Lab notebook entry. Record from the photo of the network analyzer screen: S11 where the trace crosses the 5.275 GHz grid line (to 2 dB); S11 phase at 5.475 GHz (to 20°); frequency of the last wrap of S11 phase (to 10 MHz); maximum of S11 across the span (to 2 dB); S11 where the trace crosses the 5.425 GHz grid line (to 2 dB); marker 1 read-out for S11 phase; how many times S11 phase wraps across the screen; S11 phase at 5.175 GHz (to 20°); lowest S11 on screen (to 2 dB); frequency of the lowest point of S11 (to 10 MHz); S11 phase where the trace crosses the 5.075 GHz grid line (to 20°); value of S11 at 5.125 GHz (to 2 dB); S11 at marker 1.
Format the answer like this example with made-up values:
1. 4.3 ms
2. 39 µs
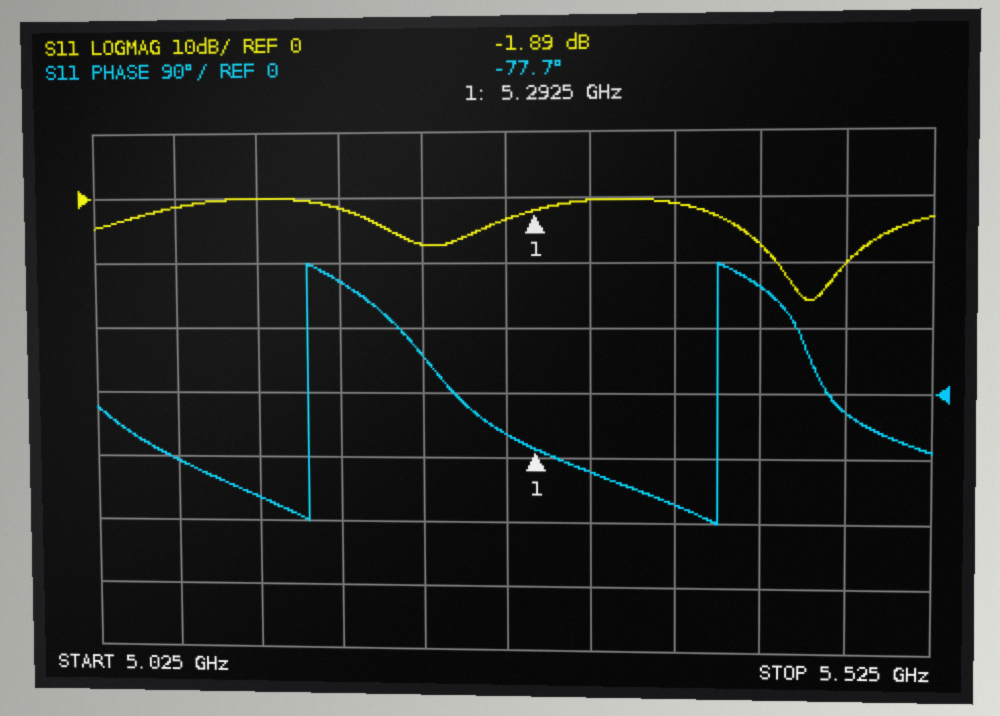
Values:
1. -4 dB
2. -20°
3. 5.40 GHz
4. 0 dB
5. -8 dB
6. -77.7°
7. 2
8. 160°
9. -16 dB
10. 5.45 GHz
11. -100°
12. 0 dB
13. -1.89 dB
